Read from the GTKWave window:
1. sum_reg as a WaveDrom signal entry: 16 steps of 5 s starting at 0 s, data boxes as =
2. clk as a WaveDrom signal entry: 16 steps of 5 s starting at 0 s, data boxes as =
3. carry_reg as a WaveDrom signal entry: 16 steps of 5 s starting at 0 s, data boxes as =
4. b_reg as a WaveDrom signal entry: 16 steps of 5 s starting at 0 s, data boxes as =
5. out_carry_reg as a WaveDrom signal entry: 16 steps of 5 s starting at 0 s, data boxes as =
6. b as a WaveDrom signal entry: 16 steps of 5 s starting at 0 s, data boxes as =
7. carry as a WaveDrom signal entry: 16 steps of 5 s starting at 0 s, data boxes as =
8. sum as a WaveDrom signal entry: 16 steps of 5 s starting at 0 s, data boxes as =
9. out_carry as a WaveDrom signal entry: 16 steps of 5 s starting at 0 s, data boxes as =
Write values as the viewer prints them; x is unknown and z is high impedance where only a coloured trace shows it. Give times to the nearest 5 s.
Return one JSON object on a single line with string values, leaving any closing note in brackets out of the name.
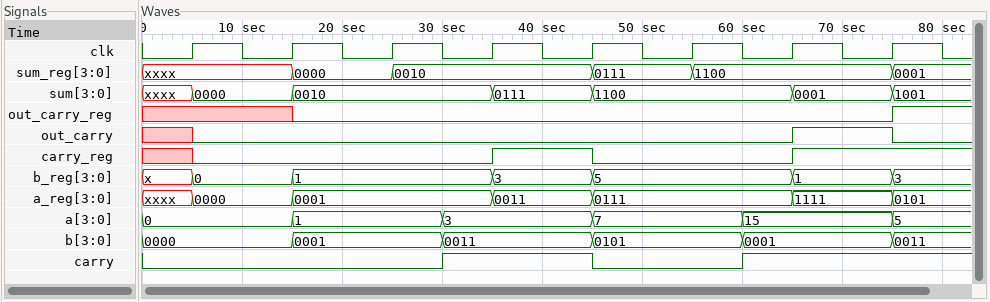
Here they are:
{"sum_reg as a WaveDrom signal entry: 16 steps of 5 s starting at 0 s, data boxes as =": "{name: 'sum_reg', wave: 'x..=.=...=.=...=', data: '0000 0010 0111 1100 0001'}", "clk as a WaveDrom signal entry: 16 steps of 5 s starting at 0 s, data boxes as =": "{name: 'clk', wave: '0101010101010101'}", "carry_reg as a WaveDrom signal entry: 16 steps of 5 s starting at 0 s, data boxes as =": "{name: 'carry_reg', wave: 'x0.....1.0...1..'}", "b_reg as a WaveDrom signal entry: 16 steps of 5 s starting at 0 s, data boxes as =": "{name: 'b_reg', wave: 'x=.=...=.=...=.=', data: '0 1 3 5 1 3'}", "out_carry_reg as a WaveDrom signal entry: 16 steps of 5 s starting at 0 s, data boxes as =": "{name: 'out_carry_reg', wave: 'x..0...........1'}", "b as a WaveDrom signal entry: 16 steps of 5 s starting at 0 s, data boxes as =": "{name: 'b', wave: '=..=..=..=..=..=', data: '0000 0001 0011 0101 0001 0011'}", "carry as a WaveDrom signal entry: 16 steps of 5 s starting at 0 s, data boxes as =": "{name: 'carry', wave: '0.....1..0..1...'}", "sum as a WaveDrom signal entry: 16 steps of 5 s starting at 0 s, data boxes as =": "{name: 'sum', wave: 'x=.=...=.=...=.=', data: '0000 0010 0111 1100 0001 1001'}", "out_carry as a WaveDrom signal entry: 16 steps of 5 s starting at 0 s, data boxes as =": "{name: 'out_carry', wave: 'x0...........1.0'}"}
